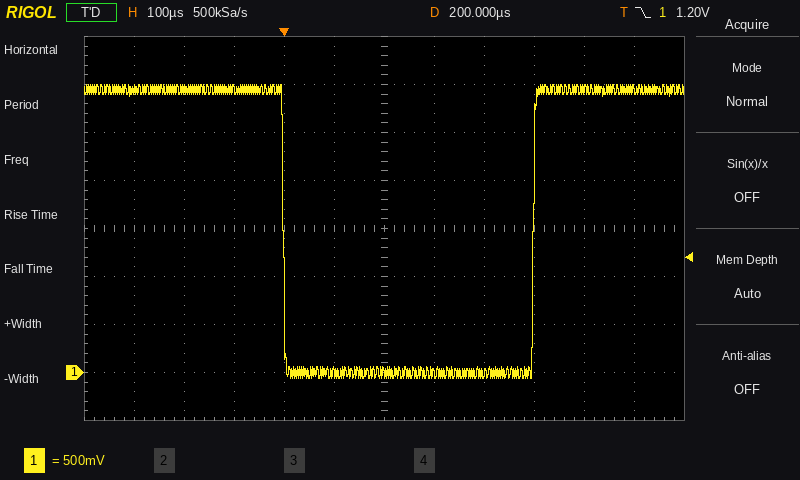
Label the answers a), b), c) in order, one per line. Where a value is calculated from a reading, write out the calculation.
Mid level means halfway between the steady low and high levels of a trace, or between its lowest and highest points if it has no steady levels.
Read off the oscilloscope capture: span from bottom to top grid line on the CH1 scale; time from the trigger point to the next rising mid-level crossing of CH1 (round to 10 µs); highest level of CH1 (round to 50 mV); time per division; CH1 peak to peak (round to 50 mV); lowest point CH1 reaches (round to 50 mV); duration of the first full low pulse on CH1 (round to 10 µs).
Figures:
a) 4 V
b) 500 µs
c) 3.00 V
d) 100 µs
e) 3.00 V − (-50 mV) = 3.05 V
f) -50 mV
g) 500 µs
